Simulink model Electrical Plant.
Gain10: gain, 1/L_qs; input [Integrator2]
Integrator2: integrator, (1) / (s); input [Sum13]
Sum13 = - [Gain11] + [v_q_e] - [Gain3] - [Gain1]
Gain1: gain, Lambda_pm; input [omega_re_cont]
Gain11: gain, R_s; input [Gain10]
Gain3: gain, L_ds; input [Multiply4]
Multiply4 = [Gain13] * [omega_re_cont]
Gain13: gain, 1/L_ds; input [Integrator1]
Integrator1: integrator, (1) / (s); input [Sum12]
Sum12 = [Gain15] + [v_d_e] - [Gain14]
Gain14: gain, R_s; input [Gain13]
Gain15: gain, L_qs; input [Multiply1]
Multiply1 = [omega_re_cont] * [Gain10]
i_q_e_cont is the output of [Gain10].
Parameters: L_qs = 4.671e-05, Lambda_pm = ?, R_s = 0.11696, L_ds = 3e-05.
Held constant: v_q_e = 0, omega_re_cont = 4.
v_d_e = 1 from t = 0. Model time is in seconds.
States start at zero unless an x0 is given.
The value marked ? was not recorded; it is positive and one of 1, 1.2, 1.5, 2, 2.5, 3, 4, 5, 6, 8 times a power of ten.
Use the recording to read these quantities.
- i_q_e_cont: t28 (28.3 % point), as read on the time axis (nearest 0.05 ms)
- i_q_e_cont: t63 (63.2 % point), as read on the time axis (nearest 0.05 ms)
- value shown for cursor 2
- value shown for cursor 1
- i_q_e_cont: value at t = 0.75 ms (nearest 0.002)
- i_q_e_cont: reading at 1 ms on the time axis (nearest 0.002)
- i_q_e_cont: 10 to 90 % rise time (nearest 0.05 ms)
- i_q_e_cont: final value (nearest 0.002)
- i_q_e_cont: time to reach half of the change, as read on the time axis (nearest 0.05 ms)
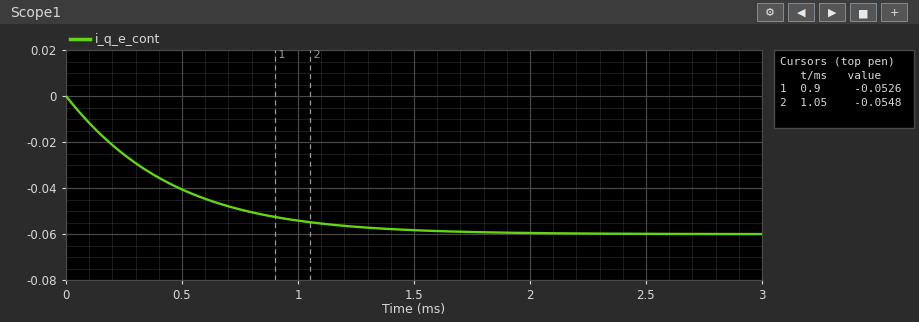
0.15 ms
0.45 ms
-0.0548
-0.0526
-0.050
-0.054
0.95 ms
-0.060
0.30 ms
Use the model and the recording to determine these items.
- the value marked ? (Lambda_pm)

0.0015
